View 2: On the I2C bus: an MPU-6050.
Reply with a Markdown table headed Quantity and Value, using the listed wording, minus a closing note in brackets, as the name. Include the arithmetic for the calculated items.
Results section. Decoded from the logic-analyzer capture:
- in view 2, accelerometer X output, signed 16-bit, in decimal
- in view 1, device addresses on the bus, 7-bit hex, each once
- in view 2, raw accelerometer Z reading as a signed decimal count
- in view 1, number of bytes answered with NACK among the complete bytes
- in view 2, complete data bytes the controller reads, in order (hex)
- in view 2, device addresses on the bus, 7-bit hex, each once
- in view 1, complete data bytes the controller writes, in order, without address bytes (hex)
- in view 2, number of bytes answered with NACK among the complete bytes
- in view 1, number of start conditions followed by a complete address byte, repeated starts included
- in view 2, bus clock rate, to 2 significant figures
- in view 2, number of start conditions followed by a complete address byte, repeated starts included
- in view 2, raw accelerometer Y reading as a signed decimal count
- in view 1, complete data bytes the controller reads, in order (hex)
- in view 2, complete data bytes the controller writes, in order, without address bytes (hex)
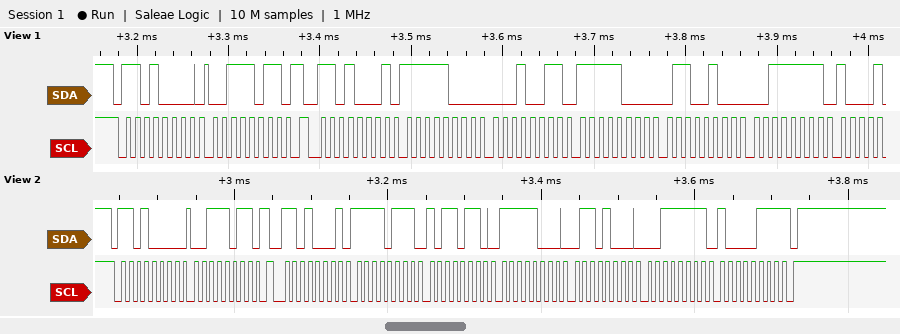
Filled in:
| Quantity | Value |
|---|---|
| in view 2, accelerometer X output, signed 16-bit, in decimal | 0xF7B6 = -2122 |
| in view 1, device addresses on the bus, 7-bit hex, each once | 0x68 |
| in view 2, raw accelerometer Z reading as a signed decimal count | 0x3F87 = 16263 |
| in view 1, number of bytes answered with NACK among the complete bytes | 0 |
| in view 2, complete data bytes the controller reads, in order | F7 B6 F8 68 3F 87 |
| in view 2, device addresses on the bus, 7-bit hex, each once | 0x68 |
| in view 1, complete data bytes the controller writes, in order, without address bytes | 3B |
| in view 2, number of bytes answered with NACK among the complete bytes | 1 |
| in view 1, number of start conditions followed by a complete address byte, repeated starts included | 2 |
| in view 2, bus clock rate, to 2 significant figures | 100 kHz |
| in view 2, number of start conditions followed by a complete address byte, repeated starts included | 2 |
| in view 2, raw accelerometer Y reading as a signed decimal count | 0xF868 = -1944 |
| in view 1, complete data bytes the controller reads, in order | F8 13 F8 64 3F |
| in view 2, complete data bytes the controller writes, in order, without address bytes | 3B |
